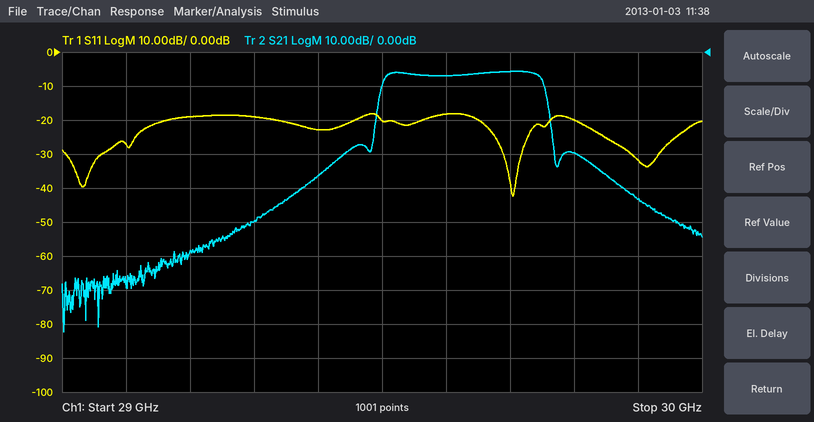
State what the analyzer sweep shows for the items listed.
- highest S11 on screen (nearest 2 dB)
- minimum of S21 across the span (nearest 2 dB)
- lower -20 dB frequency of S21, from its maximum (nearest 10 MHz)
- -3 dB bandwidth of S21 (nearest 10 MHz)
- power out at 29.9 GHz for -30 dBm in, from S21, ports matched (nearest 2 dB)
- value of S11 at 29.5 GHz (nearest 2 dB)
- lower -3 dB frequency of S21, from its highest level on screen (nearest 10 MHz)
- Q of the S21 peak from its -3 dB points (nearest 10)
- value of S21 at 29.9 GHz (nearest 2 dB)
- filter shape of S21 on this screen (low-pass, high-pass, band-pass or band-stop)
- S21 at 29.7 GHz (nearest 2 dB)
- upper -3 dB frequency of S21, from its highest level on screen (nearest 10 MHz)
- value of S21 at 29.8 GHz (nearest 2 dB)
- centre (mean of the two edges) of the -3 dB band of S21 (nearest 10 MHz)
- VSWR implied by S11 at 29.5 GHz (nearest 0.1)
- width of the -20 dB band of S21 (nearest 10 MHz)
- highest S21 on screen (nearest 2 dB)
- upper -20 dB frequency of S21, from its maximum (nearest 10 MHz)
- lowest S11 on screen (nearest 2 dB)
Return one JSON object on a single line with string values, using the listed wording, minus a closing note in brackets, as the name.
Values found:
{"highest S11 on screen": "-18 dB", "minimum of S21 across the span": "-82 dB", "lower -20 dB frequency of S21, from its maximum": "29.49 GHz", "-3 dB bandwidth of S21": "250 MHz", "power out at 29.9 GHz for -30 dBm in, from S21, ports matched": "-74 dBm", "value of S11 at 29.5 GHz": "-20 dB", "lower -3 dB frequency of S21, from its highest level on screen": "29.50 GHz", "Q of the S21 peak from its -3 dB points": "120", "value of S21 at 29.9 GHz": "-44 dB", "filter shape of S21 on this screen": "band-pass", "S21 at 29.7 GHz": "-6 dB", "upper -3 dB frequency of S21, from its highest level on screen": "29.75 GHz", "value of S21 at 29.8 GHz": "-30 dB", "centre (mean of the two edges) of the -3 dB band of S21": "29.63 GHz", "VSWR implied by S11 at 29.5 GHz": "1.2", "width of the -20 dB band of S21": "280 MHz", "highest S21 on screen": "-6 dB", "upper -20 dB frequency of S21, from its maximum": "29.77 GHz", "lowest S11 on screen": "-42 dB"}
